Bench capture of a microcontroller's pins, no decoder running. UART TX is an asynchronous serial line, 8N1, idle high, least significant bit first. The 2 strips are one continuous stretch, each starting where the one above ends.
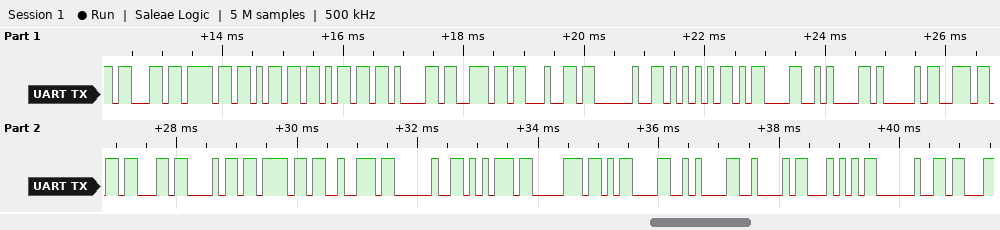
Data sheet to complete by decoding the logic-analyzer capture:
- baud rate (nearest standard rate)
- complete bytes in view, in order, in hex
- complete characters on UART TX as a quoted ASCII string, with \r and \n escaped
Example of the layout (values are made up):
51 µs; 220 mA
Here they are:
9600 baud; 63 6F 6D 6D 61 6E 64 20 55 0D 0A 41 6E 63 68 6F 72 20 75 70 0D 0A 42 54 20; "command U\r\nAnchor up\r\nBT "
